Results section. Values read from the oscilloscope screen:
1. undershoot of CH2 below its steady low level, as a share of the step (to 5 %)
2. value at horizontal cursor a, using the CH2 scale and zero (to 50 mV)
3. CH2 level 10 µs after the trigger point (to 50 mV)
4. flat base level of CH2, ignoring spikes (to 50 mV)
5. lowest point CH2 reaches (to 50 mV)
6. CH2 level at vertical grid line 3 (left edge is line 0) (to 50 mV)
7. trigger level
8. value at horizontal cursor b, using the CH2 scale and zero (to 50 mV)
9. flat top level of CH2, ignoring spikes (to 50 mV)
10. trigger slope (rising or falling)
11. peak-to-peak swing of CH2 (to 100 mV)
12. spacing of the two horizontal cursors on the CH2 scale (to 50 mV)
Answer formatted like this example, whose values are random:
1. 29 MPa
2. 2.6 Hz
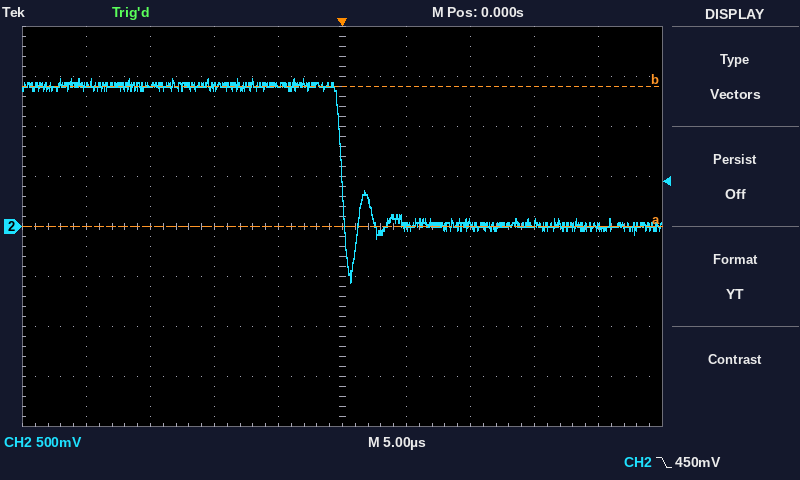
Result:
1. 40 %
2. 0 mV
3. 50 mV
4. 0 mV
5. -550 mV
6. 1.40 V
7. 450 mV
8. 1.40 V
9. 1.40 V
10. falling
11. 2.00 V
12. 1.40 V
